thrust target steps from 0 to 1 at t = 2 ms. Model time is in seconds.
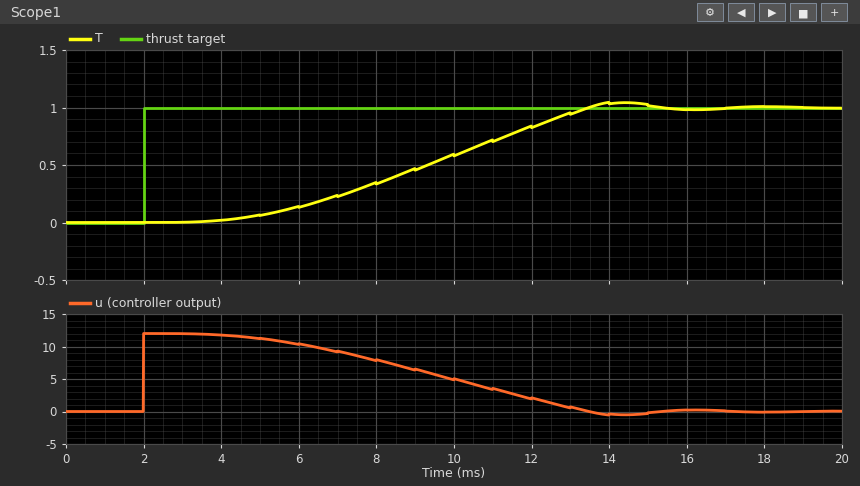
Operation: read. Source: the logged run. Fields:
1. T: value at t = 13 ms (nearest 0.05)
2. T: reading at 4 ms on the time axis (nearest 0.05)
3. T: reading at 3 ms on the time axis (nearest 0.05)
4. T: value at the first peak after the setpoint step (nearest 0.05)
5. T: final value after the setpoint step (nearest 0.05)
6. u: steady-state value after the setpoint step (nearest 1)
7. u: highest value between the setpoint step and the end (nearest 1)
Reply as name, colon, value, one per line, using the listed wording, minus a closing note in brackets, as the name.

T: value at t = 13 ms: 0.95
T: reading at 4 ms on the time axis: 0.00
T: reading at 3 ms on the time axis: 0.00
T: value at the first peak after the setpoint step: 1.05
T: final value after the setpoint step: 1.00
u: steady-state value after the setpoint step: 0
u: highest value between the setpoint step and the end: 12
